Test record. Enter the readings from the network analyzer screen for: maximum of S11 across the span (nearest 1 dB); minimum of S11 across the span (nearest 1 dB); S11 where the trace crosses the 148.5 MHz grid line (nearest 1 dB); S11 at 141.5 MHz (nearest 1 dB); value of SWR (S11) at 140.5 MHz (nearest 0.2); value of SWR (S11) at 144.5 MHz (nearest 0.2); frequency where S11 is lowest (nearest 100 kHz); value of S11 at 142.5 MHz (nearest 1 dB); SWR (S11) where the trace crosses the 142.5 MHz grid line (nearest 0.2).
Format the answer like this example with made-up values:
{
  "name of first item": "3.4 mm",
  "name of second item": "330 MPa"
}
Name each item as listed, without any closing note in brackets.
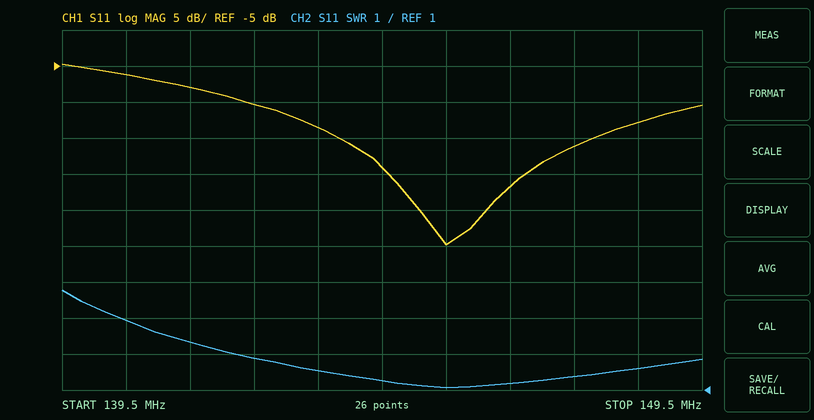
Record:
{
  "maximum of S11 across the span": "-5 dB",
  "minimum of S11 across the span": "-30 dB",
  "S11 where the trace crosses the 148.5 MHz grid line": "-13 dB",
  "S11 at 141.5 MHz": "-8 dB",
  "value of SWR (S11) at 140.5 MHz": "3.0",
  "value of SWR (S11) at 144.5 MHz": "1.2",
  "frequency where S11 is lowest": "145.5 MHz",
  "value of S11 at 142.5 MHz": "-10 dB",
  "SWR (S11) where the trace crosses the 142.5 MHz grid line": "1.8"
}
